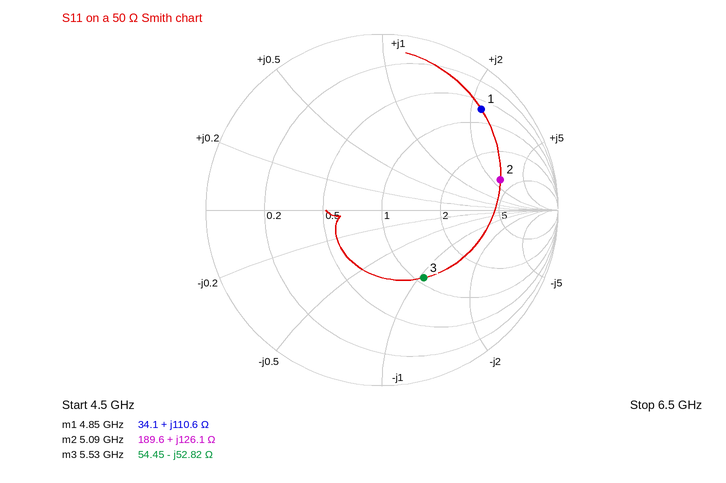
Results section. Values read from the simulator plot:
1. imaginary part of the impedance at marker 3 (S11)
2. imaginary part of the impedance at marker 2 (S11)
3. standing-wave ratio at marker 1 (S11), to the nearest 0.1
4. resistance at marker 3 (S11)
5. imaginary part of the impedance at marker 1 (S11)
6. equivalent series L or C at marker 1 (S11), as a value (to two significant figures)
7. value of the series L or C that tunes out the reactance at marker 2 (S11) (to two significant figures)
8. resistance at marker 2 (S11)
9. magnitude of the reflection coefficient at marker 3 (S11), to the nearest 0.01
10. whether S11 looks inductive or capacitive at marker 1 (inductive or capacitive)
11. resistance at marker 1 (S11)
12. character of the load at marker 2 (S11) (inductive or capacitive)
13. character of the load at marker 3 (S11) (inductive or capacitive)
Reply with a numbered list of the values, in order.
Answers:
1. -52.82 Ω
2. +126.1 Ω
3. 9.2
4. 54.45 Ω
5. +110.6 Ω
6. 3.6 nH
7. 250 fF
8. 189.6 Ω
9. 0.45
10. inductive
11. 34.1 Ω
12. inductive
13. capacitive
